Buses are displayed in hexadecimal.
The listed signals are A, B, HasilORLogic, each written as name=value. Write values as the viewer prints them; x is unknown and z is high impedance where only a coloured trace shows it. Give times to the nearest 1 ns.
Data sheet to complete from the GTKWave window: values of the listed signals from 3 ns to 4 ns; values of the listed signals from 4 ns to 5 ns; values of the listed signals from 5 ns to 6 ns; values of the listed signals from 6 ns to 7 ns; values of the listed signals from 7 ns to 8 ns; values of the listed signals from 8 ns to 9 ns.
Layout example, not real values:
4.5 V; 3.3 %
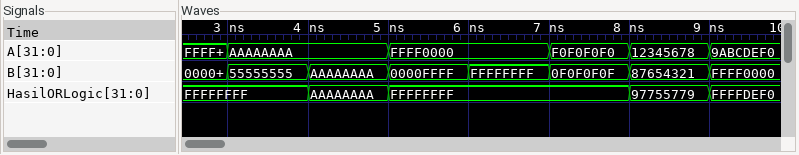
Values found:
A=AAAAAAAA, B=55555555, HasilORLogic=FFFFFFFF; A=AAAAAAAA, B=AAAAAAAA, HasilORLogic=AAAAAAAA; A=FFFF0000, B=0000FFFF, HasilORLogic=FFFFFFFF; A=FFFF0000, B=FFFFFFFF, HasilORLogic=FFFFFFFF; A=F0F0F0F0, B=0F0F0F0F, HasilORLogic=FFFFFFFF; A=12345678, B=87654321, HasilORLogic=97755779
